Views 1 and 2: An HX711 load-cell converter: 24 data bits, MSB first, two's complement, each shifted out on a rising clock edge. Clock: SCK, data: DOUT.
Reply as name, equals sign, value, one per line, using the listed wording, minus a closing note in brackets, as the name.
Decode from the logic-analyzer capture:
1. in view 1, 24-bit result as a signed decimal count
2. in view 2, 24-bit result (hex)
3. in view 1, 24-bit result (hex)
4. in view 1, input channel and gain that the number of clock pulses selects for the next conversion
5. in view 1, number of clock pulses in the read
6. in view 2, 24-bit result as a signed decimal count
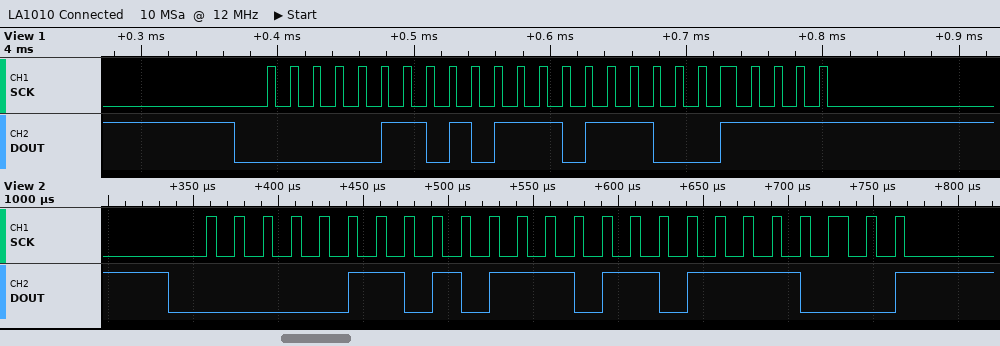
in view 1, 24-bit result as a signed decimal count = 441231
in view 2, 24-bit result = 0x06BB78
in view 1, 24-bit result = 0x06BB8F
in view 1, input channel and gain that the number of clock pulses selects for the next conversion = channel A, gain 128
in view 1, number of clock pulses in the read = 25
in view 2, 24-bit result as a signed decimal count = 441208
